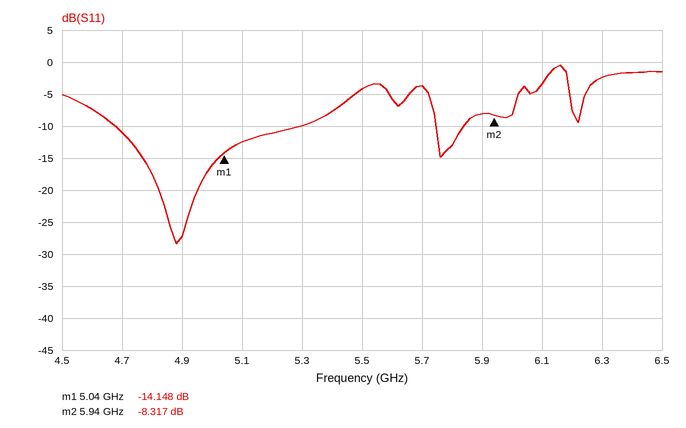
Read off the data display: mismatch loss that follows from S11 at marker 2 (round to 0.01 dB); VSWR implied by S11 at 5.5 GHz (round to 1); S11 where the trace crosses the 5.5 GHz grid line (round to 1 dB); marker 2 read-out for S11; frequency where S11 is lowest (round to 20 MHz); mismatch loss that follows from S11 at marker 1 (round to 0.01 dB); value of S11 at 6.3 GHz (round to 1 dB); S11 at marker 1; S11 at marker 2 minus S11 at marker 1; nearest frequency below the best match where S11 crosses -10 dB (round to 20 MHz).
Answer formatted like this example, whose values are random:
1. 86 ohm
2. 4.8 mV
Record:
1. 0.69 dB
2. 4
3. -4 dB
4. -8.317 dB
5. 4.88 GHz
6. 0.17 dB
7. -2 dB
8. -14.148 dB
9. 5.831 dB
10. 4.68 GHz
